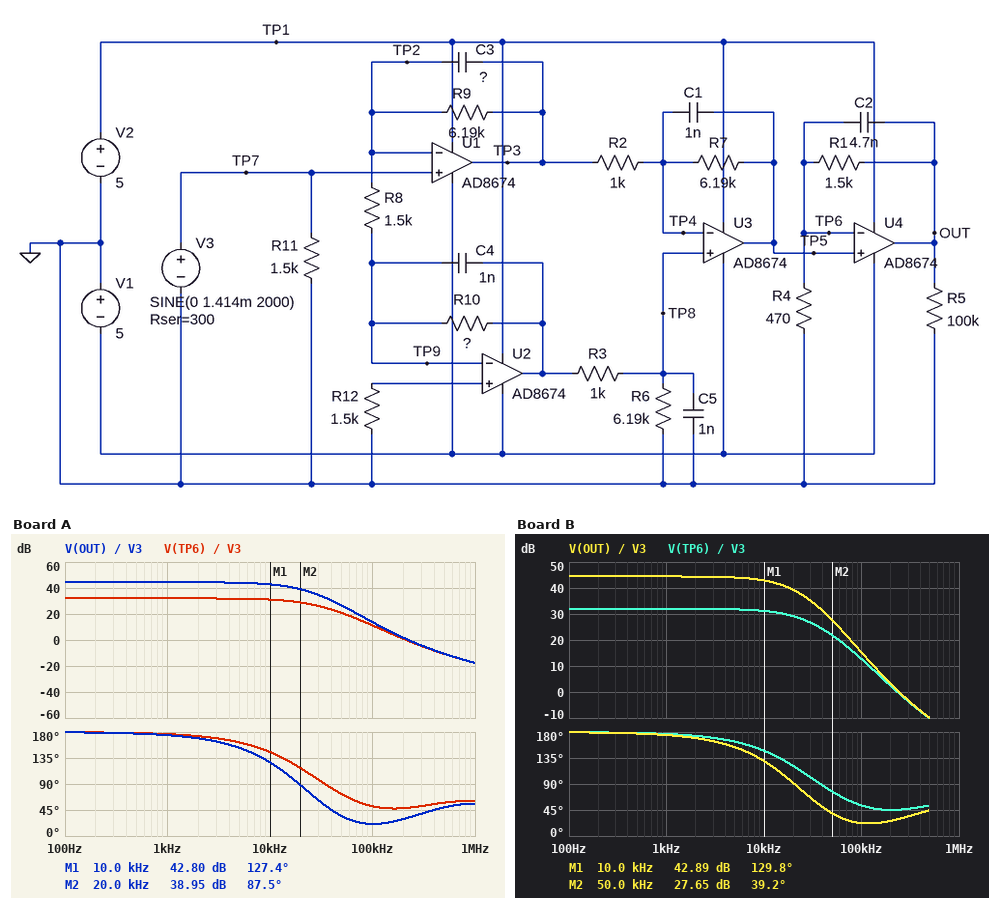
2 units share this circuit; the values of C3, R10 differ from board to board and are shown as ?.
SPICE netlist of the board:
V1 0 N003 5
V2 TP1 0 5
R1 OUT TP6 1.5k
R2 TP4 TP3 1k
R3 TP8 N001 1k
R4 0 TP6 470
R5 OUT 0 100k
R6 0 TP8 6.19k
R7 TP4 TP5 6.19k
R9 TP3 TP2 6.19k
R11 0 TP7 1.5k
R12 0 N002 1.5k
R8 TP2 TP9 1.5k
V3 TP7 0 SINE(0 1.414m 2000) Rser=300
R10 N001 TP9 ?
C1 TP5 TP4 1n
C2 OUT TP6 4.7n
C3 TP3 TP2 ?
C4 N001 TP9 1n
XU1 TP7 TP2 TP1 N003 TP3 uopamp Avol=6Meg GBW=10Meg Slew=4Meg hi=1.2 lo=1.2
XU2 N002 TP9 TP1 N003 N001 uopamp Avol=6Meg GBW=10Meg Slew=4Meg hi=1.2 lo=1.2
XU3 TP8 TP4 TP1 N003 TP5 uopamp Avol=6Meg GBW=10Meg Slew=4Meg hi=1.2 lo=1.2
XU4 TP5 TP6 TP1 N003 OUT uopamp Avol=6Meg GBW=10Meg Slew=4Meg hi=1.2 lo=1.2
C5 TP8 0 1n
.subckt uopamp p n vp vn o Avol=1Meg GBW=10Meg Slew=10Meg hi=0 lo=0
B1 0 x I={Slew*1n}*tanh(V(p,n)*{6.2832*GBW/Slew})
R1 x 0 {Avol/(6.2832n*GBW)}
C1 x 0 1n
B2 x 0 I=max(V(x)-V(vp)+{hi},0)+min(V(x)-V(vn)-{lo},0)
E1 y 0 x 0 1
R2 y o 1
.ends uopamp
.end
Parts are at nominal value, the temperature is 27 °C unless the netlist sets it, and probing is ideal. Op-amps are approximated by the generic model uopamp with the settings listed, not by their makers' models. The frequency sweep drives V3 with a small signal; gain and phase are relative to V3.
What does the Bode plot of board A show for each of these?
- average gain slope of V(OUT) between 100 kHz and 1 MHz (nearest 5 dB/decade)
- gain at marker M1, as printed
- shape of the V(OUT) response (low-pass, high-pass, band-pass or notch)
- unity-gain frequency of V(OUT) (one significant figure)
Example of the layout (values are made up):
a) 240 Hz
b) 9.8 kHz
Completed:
a) -30 dB/decade
b) 42.80 dB
c) low-pass
d) 200 kHz
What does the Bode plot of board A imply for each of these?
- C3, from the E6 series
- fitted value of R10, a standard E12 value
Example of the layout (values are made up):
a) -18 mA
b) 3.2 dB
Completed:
a) 680 pF
b) 3.9 kΩ
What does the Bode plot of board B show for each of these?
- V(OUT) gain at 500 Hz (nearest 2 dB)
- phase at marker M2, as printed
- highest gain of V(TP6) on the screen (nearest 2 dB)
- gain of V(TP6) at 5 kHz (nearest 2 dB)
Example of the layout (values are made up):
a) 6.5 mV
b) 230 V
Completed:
a) 44 dB
b) 39.2 deg
c) 32 dB
d) 32 dB
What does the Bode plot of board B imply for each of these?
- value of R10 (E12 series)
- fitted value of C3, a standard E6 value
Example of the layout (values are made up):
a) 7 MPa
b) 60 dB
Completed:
a) 3.9 kΩ
b) 470 pF
